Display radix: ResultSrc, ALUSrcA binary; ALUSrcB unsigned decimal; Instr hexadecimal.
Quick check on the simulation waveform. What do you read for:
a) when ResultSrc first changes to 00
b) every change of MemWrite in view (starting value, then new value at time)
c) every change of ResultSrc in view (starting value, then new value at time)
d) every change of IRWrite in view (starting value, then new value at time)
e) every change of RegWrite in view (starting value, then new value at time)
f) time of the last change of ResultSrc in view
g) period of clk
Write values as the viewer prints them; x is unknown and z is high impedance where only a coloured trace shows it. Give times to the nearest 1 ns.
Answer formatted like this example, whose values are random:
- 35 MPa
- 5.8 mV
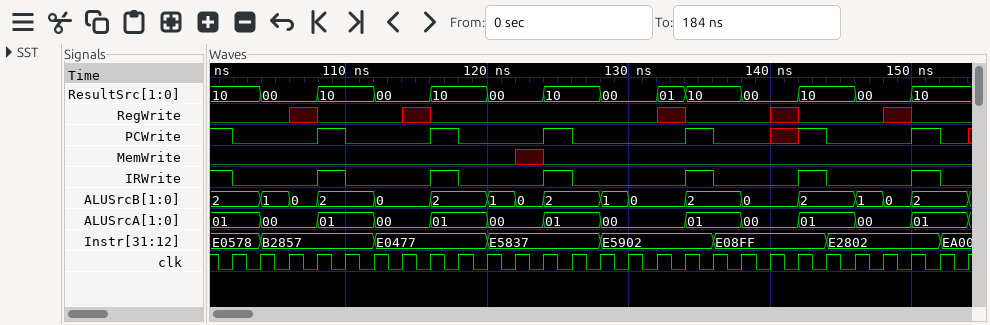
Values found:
- 104 ns
- 0, x at 122 ns, 0 at 124 ns
- 10, 00 at 104 ns, 10 at 108 ns, 00 at 112 ns, 10 at 116 ns, 00 at 120 ns, 10 at 124 ns, 00 at 128 ns, 01 at 132 ns, 10 at 134 ns, 00 at 138 ns, 10 at 142 ns, 00 at 146 ns, 10 at 150 ns
- 1, 0 at 102 ns, 1 at 108 ns, 0 at 110 ns, 1 at 116 ns, 0 at 118 ns, 1 at 124 ns, 0 at 126 ns, 1 at 134 ns, 0 at 136 ns, 1 at 142 ns, 0 at 144 ns, 1 at 150 ns, 0 at 152 ns
- 0, x at 106 ns, 0 at 108 ns, x at 114 ns, 0 at 116 ns, x at 132 ns, 0 at 134 ns, x at 140 ns, 0 at 142 ns, x at 148 ns, 0 at 150 ns
- 150 ns
- 2 ns
